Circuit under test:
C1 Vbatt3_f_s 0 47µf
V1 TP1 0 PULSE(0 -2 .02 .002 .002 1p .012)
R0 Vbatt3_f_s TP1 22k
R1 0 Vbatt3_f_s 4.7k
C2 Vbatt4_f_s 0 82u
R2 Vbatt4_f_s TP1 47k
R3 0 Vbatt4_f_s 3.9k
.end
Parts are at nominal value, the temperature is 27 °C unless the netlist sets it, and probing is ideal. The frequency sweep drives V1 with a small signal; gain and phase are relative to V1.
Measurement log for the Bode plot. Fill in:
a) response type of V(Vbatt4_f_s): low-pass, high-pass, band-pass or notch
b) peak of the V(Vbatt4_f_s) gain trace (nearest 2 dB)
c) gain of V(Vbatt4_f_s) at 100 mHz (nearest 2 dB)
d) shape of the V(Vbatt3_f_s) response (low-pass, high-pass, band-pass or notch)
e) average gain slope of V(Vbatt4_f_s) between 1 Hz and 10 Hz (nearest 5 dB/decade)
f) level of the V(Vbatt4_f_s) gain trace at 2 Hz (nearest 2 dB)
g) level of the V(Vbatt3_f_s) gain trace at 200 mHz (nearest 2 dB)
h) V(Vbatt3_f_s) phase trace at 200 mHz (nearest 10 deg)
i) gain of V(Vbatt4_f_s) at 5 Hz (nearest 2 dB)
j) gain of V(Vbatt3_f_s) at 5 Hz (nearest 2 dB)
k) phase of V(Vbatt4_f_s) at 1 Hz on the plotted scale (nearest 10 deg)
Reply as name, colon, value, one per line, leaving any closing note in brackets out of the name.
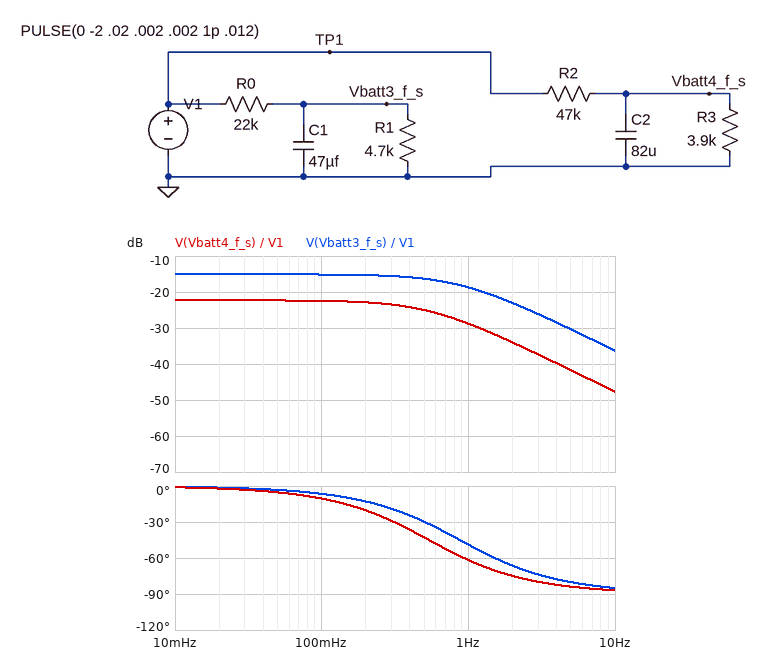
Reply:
response type of V(Vbatt4_f_s): low-pass, high-pass, band-pass or notch: low-pass
peak of the V(Vbatt4_f_s) gain trace: -22 dB
gain of V(Vbatt4_f_s) at 100 mHz: -22 dB
shape of the V(Vbatt3_f_s) response: low-pass
average gain slope of V(Vbatt4_f_s) between 1 Hz and 10 Hz: -20 dB/decade
level of the V(Vbatt4_f_s) gain trace at 2 Hz: -34 dB
level of the V(Vbatt3_f_s) gain trace at 200 mHz: -16 dB
V(Vbatt3_f_s) phase trace at 200 mHz: -10 deg
gain of V(Vbatt4_f_s) at 5 Hz: -42 dB
gain of V(Vbatt3_f_s) at 5 Hz: -30 dB
phase of V(Vbatt4_f_s) at 1 Hz on the plotted scale: -60 deg
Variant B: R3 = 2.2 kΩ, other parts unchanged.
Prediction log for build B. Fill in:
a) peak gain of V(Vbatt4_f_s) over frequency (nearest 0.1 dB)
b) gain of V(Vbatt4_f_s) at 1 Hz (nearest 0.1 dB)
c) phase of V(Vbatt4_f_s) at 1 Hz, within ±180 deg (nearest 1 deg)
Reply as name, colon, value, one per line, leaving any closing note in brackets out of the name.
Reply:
peak gain of V(Vbatt4_f_s) over frequency: -27.0 dB
gain of V(Vbatt4_f_s) at 1 Hz: -30.4 dB
phase of V(Vbatt4_f_s) at 1 Hz, within ±180 deg: -47 deg
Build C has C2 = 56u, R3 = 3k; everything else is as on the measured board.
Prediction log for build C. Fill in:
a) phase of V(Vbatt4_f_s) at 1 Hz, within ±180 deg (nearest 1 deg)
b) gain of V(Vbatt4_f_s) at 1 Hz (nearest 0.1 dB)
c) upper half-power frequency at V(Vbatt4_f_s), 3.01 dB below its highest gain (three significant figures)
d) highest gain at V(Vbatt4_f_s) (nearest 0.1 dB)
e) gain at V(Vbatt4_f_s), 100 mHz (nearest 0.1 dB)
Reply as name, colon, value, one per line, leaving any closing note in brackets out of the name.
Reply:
phase of V(Vbatt4_f_s) at 1 Hz, within ±180 deg: -45 deg
gain of V(Vbatt4_f_s) at 1 Hz: -27.4 dB
upper half-power frequency at V(Vbatt4_f_s), 3.01 dB below its highest gain: 1.01 Hz
highest gain at V(Vbatt4_f_s): -24.4 dB
gain at V(Vbatt4_f_s), 100 mHz: -24.5 dB
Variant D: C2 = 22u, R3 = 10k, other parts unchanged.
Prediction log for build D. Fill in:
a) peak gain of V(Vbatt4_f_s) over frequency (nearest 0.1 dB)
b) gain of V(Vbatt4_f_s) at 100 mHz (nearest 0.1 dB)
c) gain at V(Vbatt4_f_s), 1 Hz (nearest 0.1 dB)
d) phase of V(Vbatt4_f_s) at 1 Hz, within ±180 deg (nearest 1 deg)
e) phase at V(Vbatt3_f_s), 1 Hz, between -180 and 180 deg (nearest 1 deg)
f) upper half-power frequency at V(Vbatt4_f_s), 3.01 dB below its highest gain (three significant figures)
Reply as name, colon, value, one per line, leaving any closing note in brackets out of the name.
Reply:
peak gain of V(Vbatt4_f_s) over frequency: -15.1 dB
gain of V(Vbatt4_f_s) at 100 mHz: -15.2 dB
gain at V(Vbatt4_f_s), 1 Hz: -18.7 dB
phase of V(Vbatt4_f_s) at 1 Hz, within ±180 deg: -49 deg
phase at V(Vbatt3_f_s), 1 Hz, between -180 and 180 deg: -49 deg
upper half-power frequency at V(Vbatt4_f_s), 3.01 dB below its highest gain: 877 mHz
